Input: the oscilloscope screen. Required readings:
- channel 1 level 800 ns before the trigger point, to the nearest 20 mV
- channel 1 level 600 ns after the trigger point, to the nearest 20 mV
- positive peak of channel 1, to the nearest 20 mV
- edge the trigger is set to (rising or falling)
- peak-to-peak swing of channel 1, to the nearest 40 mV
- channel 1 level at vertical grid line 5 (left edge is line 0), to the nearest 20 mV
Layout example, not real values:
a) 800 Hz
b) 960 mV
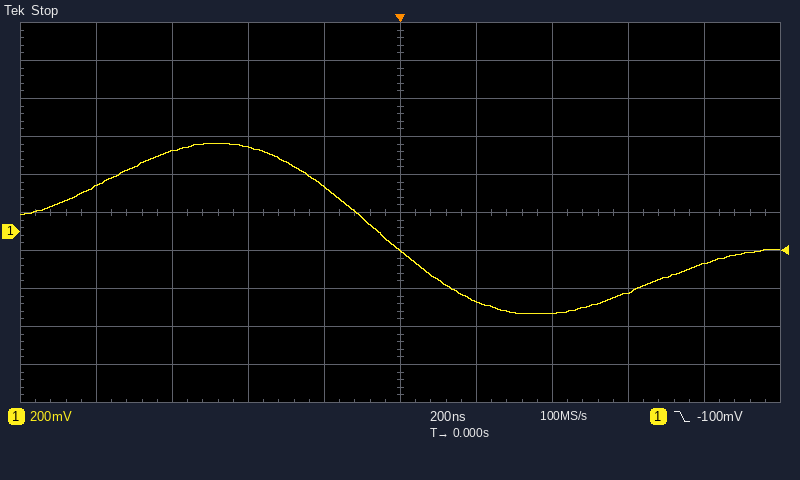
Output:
a) 240 mV
b) -320 mV
c) 460 mV
d) falling
e) 880 mV
f) -100 mV
